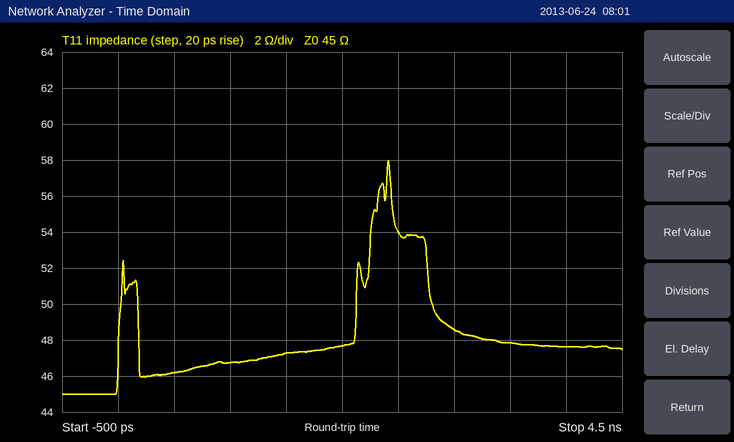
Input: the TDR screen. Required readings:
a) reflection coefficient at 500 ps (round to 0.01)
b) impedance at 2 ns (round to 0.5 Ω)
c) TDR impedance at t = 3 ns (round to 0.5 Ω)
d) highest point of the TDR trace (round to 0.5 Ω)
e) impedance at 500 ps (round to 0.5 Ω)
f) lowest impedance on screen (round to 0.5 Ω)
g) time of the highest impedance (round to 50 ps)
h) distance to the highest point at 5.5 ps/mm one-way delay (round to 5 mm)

+0.01
47.5 Ω
48.5 Ω
58.0 Ω
46.0 Ω
45.0 Ω
2.40 ns
220 mm
